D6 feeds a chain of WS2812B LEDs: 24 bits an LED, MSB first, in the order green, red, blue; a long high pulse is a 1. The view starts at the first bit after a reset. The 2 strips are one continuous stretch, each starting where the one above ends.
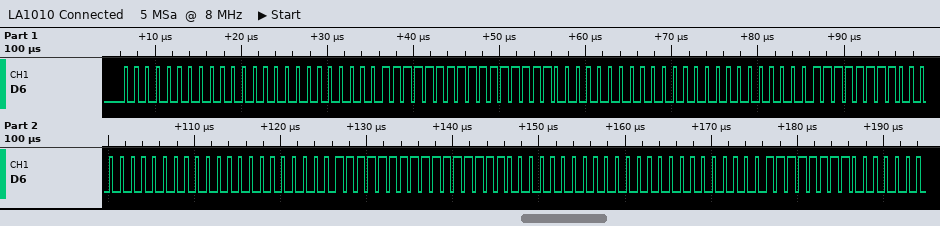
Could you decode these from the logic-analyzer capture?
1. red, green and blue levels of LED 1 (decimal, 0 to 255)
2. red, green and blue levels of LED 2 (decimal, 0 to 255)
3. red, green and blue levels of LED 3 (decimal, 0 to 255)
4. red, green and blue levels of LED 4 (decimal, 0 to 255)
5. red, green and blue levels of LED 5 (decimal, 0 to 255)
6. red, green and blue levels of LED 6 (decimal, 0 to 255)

0, 0, 0
255, 255, 0
0, 0, 255
0, 0, 0
255, 255, 0
0, 0, 255
